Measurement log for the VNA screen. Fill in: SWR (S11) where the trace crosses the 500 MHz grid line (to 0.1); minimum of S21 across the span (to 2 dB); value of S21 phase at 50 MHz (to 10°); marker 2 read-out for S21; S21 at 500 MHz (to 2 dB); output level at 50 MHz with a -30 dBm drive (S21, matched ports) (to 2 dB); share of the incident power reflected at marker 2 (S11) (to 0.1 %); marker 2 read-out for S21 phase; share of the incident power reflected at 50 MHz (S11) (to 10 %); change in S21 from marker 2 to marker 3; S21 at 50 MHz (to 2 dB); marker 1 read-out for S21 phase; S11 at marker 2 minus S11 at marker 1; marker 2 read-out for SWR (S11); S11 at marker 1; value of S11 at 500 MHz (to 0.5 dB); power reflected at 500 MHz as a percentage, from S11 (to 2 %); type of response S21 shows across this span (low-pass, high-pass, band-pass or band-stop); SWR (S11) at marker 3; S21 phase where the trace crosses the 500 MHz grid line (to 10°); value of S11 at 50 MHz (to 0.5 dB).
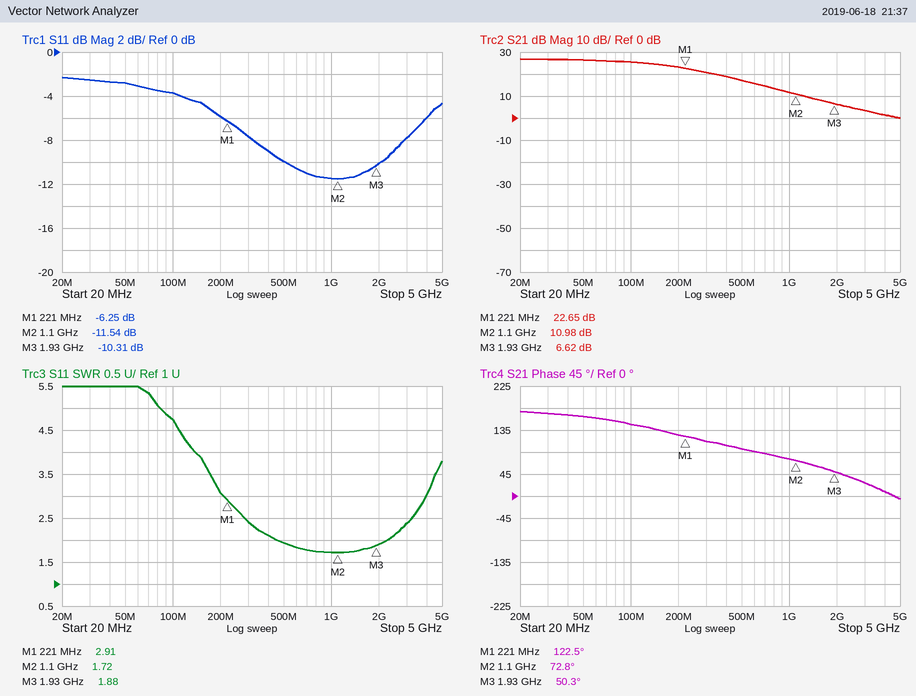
1.9
0 dB
160°
10.98 dB
18 dB
-4 dBm
7.0 %
72.8°
50 %
-4.36 dB
26 dB
122.5°
-5.29 dB
1.72
-6.25 dB
-10.0 dB
10 %
low-pass
1.88
100°
-3.0 dB
